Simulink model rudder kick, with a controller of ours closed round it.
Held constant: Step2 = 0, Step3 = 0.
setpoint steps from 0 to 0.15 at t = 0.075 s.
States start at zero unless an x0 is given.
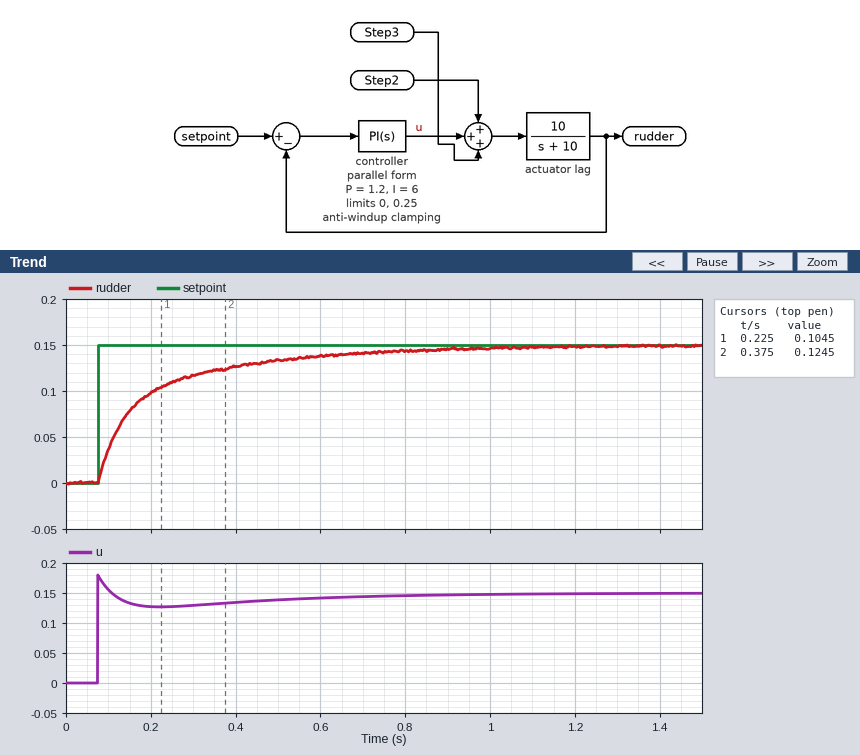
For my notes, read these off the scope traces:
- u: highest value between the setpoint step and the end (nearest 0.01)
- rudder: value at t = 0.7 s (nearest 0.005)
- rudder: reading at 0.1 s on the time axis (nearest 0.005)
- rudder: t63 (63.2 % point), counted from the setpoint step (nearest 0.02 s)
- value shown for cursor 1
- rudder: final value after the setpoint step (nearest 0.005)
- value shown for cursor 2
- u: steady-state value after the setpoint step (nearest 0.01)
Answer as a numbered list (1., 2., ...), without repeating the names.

1. 0.18
2. 0.140
3. 0.035
4. 0.12 s
5. 0.1045
6. 0.150
7. 0.1245
8. 0.15
